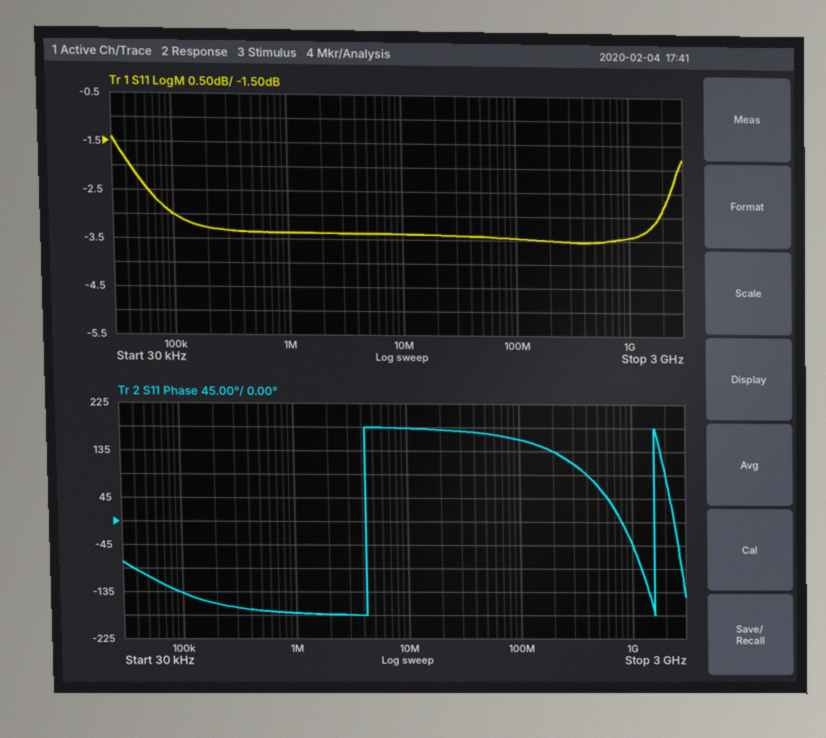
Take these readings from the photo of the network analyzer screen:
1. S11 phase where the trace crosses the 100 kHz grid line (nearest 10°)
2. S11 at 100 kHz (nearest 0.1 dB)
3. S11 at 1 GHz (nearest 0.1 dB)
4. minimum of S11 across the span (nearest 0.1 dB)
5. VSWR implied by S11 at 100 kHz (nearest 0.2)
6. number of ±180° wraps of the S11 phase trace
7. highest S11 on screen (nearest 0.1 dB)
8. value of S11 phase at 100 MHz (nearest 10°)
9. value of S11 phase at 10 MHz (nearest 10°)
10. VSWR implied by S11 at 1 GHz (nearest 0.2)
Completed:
-140°
-3.0 dB
-3.4 dB
-3.5 dB
5.8
2
-1.4 dB
160°
180°
5.2
